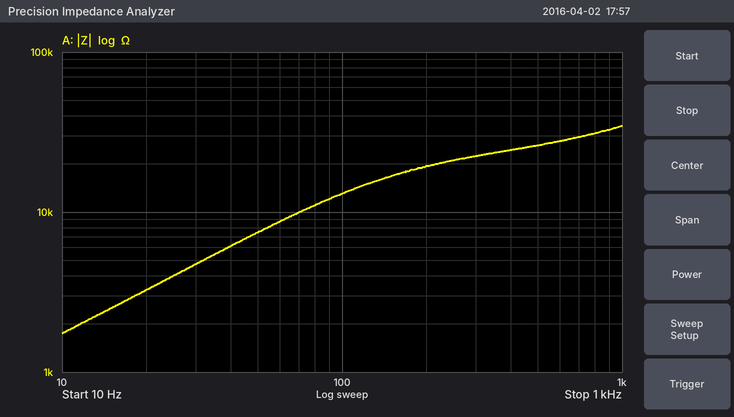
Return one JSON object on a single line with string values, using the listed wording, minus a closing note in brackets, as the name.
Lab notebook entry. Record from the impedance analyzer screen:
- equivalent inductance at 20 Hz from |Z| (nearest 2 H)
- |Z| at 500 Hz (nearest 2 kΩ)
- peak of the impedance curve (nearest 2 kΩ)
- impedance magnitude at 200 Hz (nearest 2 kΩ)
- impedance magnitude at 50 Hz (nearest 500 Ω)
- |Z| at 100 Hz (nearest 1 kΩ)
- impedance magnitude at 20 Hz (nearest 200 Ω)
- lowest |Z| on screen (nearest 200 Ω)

{"equivalent inductance at 20 Hz from |Z|": "26 H", "|Z| at 500 Hz": "26 kΩ", "peak of the impedance curve": "34 kΩ", "impedance magnitude at 200 Hz": "20 kΩ", "impedance magnitude at 50 Hz": "7.5 kΩ", "|Z| at 100 Hz": "13 kΩ", "impedance magnitude at 20 Hz": "3.2 kΩ", "lowest |Z| on screen": "1.8 kΩ"}
